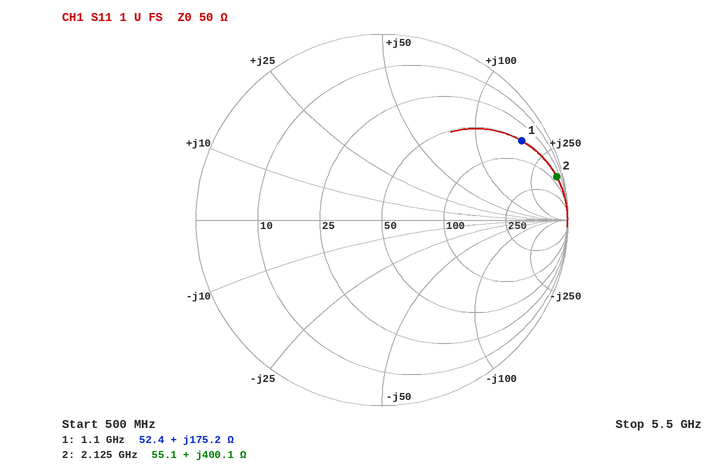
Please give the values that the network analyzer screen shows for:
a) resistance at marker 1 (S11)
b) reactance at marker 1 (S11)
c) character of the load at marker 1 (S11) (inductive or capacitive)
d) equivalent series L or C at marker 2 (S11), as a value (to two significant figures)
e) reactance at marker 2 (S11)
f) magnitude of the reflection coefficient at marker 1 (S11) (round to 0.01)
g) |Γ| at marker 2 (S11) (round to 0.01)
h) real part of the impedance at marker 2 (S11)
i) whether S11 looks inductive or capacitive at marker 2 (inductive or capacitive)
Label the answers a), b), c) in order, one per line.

a) 52.4 Ω
b) +175.2 Ω
c) inductive
d) 30 nH
e) +400.1 Ω
f) 0.86
g) 0.97
h) 55.1 Ω
i) inductive
